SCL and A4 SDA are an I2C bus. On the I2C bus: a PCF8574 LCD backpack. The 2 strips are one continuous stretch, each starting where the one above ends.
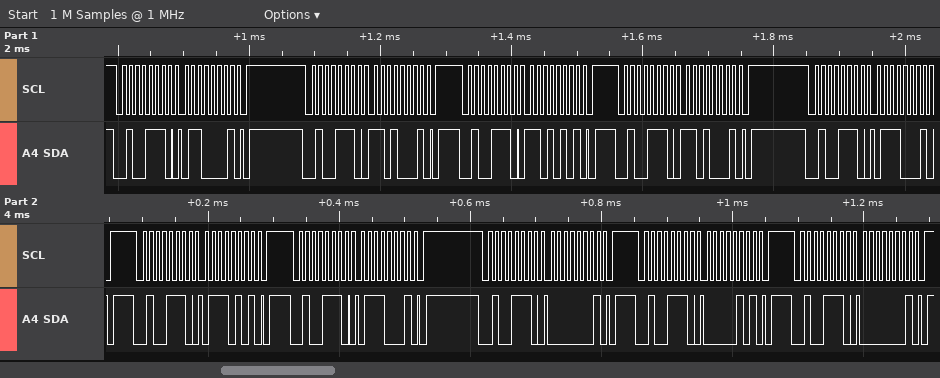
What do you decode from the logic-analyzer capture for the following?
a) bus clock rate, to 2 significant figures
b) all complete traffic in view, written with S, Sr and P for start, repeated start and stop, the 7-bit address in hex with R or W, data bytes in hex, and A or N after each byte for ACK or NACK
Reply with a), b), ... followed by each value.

a) 100 kHz
b) S 27W A 61 A P S 27W A D1 A P S 27W A D5 A P S 27W A D1 A P S 27W A 71 A P S 27W A 75 A P S 27W A 71 A P S 27W A 01 A P S 27W A 05 A P S 27W A 01 A P
